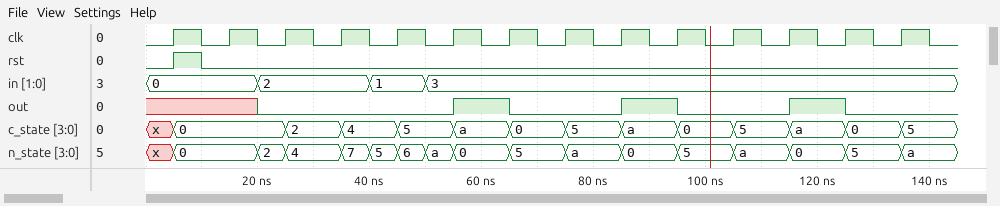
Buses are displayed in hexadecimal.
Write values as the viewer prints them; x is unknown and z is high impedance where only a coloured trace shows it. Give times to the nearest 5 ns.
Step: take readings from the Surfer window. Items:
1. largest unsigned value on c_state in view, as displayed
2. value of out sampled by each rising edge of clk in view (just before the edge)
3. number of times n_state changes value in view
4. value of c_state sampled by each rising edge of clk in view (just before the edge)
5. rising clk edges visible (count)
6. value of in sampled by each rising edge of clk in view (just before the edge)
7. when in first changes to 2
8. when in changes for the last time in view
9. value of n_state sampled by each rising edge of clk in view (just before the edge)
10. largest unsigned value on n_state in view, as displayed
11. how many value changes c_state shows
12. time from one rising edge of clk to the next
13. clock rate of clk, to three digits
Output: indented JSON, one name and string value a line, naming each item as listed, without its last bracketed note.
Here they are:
{
  "largest unsigned value on c_state in view, as displayed": "a",
  "value of out sampled by each rising edge of clk in view": "x x 0 0 0 0 1 0 0 1 0 0 1 0",
  "number of times n_state changes value in view": "16",
  "value of c_state sampled by each rising edge of clk in view": "x, 0, 0, 2, 4, 5, a, 0, 5, a, 0, 5, a, 0",
  "rising clk edges visible": "14",
  "value of in sampled by each rising edge of clk in view": "0, 0, 2, 2, 1, 3, 3, 3, 3, 3, 3, 3, 3, 3",
  "when in first changes to 2": "20 ns",
  "when in changes for the last time in view": "50 ns",
  "value of n_state sampled by each rising edge of clk in view": "x, 0, 2, 4, 5, a, 0, 5, a, 0, 5, a, 0, 5",
  "largest unsigned value on n_state in view, as displayed": "a",
  "how many value changes c_state shows": "13",
  "time from one rising edge of clk to the next": "10 ns",
  "clock rate of clk, to three digits": "100 MHz"
}
